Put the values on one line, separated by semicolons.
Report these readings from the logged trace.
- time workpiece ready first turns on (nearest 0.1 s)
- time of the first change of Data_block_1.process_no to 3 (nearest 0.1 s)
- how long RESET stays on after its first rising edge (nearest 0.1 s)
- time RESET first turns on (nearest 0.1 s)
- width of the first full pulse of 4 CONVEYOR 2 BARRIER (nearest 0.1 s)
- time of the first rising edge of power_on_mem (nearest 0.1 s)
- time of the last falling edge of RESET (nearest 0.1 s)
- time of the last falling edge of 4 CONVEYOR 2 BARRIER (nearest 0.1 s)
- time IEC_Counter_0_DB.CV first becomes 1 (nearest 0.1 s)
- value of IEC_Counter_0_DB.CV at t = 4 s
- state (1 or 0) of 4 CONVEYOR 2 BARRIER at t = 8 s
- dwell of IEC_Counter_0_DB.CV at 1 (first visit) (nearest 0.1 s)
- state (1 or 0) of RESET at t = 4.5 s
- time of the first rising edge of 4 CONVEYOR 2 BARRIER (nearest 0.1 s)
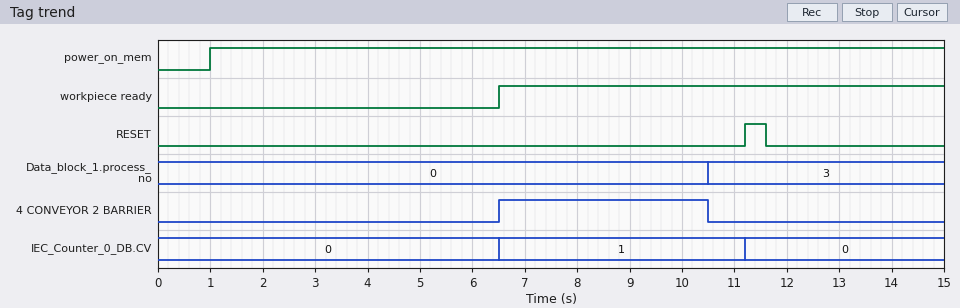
6.5 s; 10.5 s; 0.4 s; 11.2 s; 4.0 s; 1.0 s; 11.6 s; 10.5 s; 6.5 s; 0; 1; 4.7 s; 0; 6.5 s
